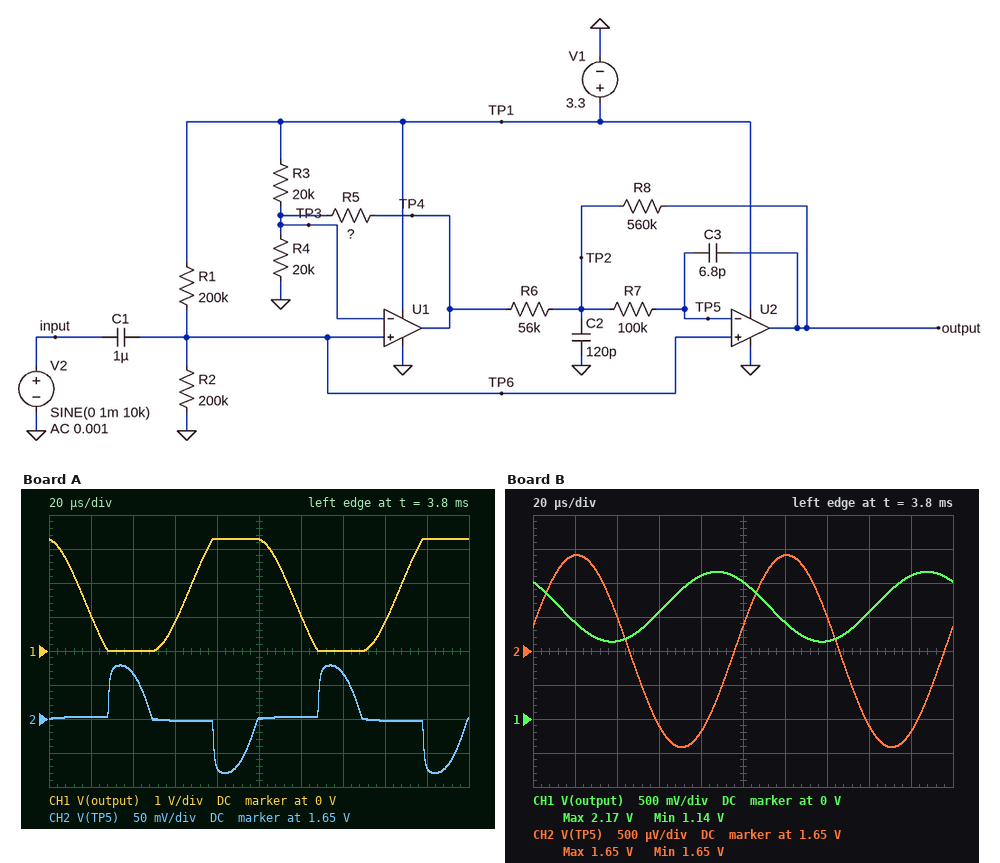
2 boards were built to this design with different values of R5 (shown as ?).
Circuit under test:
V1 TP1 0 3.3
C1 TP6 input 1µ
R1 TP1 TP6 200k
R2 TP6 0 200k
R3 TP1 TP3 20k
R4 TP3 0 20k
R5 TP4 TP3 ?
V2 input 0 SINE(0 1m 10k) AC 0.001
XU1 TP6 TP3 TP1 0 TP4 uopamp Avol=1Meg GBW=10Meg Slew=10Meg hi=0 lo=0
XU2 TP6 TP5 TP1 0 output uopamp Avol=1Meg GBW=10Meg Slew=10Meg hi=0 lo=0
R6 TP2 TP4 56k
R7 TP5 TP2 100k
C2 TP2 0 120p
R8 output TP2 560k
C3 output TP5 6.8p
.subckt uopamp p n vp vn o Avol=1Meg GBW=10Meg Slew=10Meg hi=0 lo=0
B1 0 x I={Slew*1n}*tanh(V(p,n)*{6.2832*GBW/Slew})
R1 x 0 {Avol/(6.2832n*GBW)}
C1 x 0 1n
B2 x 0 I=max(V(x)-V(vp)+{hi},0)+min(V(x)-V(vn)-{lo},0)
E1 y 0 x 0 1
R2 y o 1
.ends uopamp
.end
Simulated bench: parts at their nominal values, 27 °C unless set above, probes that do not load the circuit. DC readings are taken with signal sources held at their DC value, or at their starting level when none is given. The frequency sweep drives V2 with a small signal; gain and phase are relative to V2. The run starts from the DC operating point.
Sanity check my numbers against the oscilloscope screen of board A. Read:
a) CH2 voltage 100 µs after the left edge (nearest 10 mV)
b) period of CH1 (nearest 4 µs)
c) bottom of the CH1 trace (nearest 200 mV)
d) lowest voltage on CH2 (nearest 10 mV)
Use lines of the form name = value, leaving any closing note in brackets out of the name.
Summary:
CH2 voltage 100 µs after the left edge = 1.65 V
period of CH1 = 100 µs
bottom of the CH1 trace = 0 V
lowest voltage on CH2 = 1.57 V
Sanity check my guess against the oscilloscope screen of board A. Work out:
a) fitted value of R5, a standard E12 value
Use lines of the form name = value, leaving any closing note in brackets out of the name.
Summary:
fitted value of R5, a standard E12 value = 2.7 MΩ
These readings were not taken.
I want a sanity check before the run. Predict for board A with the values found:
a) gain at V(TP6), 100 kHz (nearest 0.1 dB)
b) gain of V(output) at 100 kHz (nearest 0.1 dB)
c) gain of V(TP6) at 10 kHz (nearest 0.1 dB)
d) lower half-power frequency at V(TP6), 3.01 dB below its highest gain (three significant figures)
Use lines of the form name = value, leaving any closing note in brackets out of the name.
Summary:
gain at V(TP6), 100 kHz = 0 dB
gain of V(output) at 100 kHz = 34.4 dB
gain of V(TP6) at 10 kHz = 0 dB
lower half-power frequency at V(TP6), 3.01 dB below its highest gain = 1.59 Hz
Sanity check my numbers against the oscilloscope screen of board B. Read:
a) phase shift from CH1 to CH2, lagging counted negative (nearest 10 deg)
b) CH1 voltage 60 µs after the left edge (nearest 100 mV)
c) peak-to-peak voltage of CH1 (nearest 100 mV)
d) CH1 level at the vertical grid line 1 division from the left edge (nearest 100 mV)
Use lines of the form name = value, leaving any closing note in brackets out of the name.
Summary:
phase shift from CH1 to CH2, lagging counted negative = -120 deg
CH1 voltage 60 µs after the left edge = 1.6 V
peak-to-peak voltage of CH1 = 1.0 V
CH1 level at the vertical grid line 1 division from the left edge = 1.4 V
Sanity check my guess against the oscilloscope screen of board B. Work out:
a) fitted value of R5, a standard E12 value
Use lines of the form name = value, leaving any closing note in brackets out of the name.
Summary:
fitted value of R5, a standard E12 value = 560 kΩ
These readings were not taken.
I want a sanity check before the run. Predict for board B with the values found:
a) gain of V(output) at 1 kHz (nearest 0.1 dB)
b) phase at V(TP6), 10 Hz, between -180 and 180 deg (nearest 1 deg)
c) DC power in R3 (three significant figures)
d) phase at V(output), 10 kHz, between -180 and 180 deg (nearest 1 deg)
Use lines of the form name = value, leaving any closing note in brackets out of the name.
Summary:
gain of V(output) at 1 kHz = 54.9 dB
phase at V(TP6), 10 Hz, between -180 and 180 deg = 9 deg
DC power in R3 = 136 µW
phase at V(output), 10 kHz, between -180 and 180 deg = 135 deg
